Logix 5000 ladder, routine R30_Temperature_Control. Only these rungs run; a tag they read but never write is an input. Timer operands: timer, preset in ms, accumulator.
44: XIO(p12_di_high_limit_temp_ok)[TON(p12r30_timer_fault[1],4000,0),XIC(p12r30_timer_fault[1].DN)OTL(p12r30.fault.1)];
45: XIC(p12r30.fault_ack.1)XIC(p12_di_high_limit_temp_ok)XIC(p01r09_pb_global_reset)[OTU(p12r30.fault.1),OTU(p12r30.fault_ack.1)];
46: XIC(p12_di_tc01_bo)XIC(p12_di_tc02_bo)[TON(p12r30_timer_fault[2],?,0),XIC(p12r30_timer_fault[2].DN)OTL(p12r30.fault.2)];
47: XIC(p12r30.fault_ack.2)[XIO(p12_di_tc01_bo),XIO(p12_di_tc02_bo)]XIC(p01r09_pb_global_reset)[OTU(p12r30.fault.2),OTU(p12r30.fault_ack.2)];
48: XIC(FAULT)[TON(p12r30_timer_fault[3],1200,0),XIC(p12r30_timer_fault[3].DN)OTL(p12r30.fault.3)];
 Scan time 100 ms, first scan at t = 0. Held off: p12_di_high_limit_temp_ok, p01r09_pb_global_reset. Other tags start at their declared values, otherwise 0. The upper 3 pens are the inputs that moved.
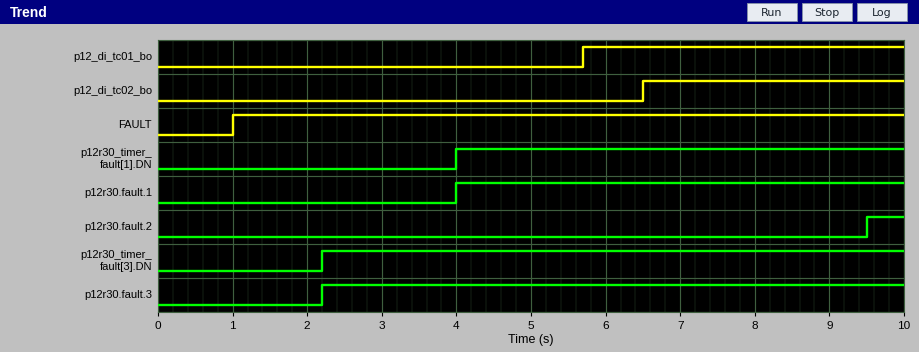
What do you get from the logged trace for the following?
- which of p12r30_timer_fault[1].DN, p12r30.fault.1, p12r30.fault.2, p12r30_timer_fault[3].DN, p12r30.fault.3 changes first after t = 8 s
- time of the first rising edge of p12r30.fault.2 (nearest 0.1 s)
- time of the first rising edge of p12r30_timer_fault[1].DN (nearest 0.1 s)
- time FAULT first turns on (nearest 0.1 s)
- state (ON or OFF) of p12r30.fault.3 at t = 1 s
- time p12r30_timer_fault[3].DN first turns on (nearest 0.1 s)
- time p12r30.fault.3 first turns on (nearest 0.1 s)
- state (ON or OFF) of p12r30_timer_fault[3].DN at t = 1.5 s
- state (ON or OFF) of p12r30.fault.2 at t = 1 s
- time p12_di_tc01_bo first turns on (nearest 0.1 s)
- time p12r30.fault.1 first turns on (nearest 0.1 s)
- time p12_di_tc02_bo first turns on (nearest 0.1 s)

p12r30.fault.2
9.5 s
4.0 s
1.0 s
OFF
2.2 s
2.2 s
OFF
OFF
5.7 s
4.0 s
6.5 s
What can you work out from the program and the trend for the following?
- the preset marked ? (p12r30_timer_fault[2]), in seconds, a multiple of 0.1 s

3.0 s
